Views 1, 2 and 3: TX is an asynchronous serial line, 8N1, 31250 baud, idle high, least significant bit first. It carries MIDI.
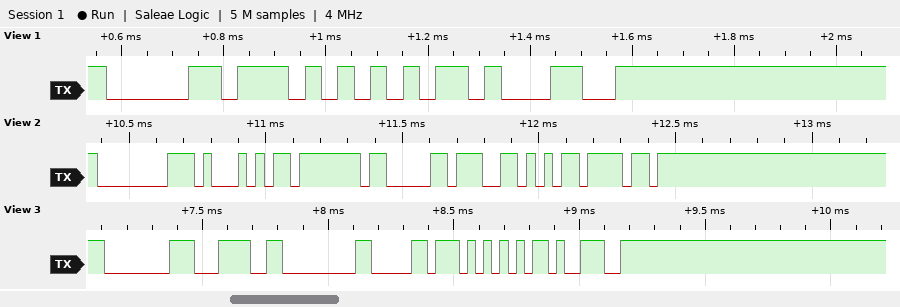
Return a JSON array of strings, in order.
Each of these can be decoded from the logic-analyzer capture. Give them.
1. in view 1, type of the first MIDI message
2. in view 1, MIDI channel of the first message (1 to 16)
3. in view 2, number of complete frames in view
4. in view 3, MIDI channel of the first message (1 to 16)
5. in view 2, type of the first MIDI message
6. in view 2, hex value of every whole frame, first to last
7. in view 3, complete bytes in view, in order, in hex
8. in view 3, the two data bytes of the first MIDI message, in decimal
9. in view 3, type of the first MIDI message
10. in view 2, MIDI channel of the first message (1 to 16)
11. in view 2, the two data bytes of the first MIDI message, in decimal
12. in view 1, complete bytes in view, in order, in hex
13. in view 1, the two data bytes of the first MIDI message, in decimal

["Control Change", "1", "6", "1", "Note Off", "0x80 0x51 0x7F 0xB0 0x56 0x6F", "80 3C 00 B0 55 39", "60, 0", "Note Off", "1", "81, 127", "B0 55 31", "85, 49"]
